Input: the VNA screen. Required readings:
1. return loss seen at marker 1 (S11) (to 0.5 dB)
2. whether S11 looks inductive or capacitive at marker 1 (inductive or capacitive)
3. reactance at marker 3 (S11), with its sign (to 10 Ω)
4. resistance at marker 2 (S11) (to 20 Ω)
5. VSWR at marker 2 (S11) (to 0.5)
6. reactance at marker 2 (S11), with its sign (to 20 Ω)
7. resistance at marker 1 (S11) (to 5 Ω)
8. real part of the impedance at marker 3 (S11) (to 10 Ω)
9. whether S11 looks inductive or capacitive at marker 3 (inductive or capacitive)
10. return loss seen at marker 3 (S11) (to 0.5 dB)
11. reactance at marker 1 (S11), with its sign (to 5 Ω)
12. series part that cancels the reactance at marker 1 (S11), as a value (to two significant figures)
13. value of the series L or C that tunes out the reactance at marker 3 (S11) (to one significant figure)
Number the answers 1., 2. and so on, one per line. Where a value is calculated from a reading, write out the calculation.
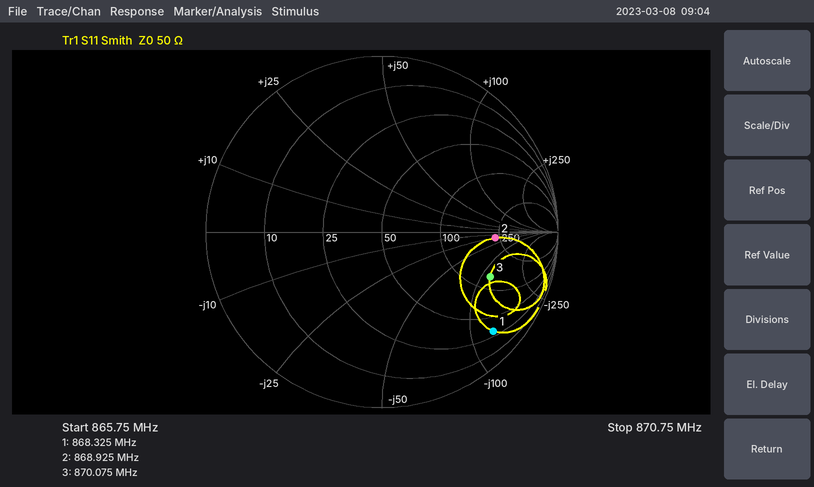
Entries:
1. 1.5 dB
2. capacitive
3. -120 Ω
4. 220 Ω
5. 4.5
6. -20 Ω
7. 30 Ω
8. 130 Ω
9. capacitive
10. 3.5 dB
11. -125 Ω
12. L = 125 Ω/(2π × 868.325 MHz) ≈ 23 nH
13. L = 120 Ω/(2π × 870.075 MHz) ≈ 22.0 nH, so 20 nH to one significant figure
